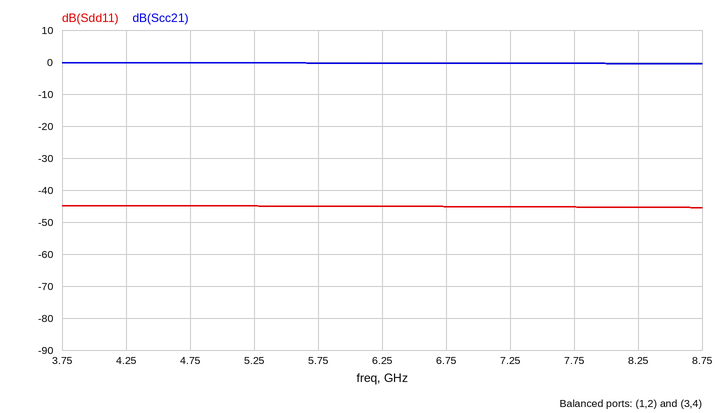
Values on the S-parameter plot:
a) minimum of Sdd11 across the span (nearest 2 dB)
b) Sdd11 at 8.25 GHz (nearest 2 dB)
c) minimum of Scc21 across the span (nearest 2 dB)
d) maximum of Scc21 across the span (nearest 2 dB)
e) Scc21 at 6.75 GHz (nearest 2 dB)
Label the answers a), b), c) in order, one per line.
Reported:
a) -46 dB
b) -46 dB
c) 0 dB
d) 0 dB
e) 0 dB
